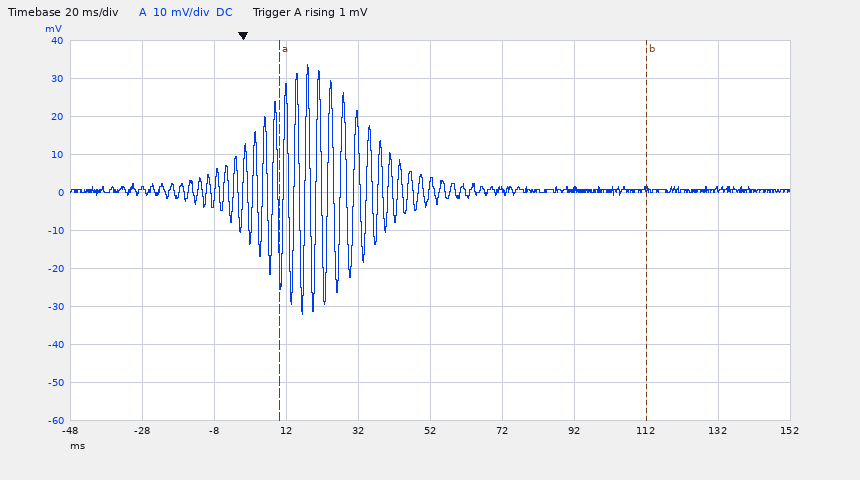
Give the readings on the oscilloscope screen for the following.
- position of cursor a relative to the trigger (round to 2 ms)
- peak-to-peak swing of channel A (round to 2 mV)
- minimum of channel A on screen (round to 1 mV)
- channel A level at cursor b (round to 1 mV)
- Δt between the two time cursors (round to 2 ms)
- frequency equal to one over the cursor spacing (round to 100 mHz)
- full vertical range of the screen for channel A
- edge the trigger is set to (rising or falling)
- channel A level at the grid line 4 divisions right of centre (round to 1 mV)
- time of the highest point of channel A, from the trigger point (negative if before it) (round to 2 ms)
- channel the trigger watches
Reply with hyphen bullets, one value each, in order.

- +10 ms
- 66 mV
- -32 mV
- 1 mV
- 102 ms
- 9.8 Hz
- 100 mV
- rising
- 1 mV
- +18 ms
- channel A
